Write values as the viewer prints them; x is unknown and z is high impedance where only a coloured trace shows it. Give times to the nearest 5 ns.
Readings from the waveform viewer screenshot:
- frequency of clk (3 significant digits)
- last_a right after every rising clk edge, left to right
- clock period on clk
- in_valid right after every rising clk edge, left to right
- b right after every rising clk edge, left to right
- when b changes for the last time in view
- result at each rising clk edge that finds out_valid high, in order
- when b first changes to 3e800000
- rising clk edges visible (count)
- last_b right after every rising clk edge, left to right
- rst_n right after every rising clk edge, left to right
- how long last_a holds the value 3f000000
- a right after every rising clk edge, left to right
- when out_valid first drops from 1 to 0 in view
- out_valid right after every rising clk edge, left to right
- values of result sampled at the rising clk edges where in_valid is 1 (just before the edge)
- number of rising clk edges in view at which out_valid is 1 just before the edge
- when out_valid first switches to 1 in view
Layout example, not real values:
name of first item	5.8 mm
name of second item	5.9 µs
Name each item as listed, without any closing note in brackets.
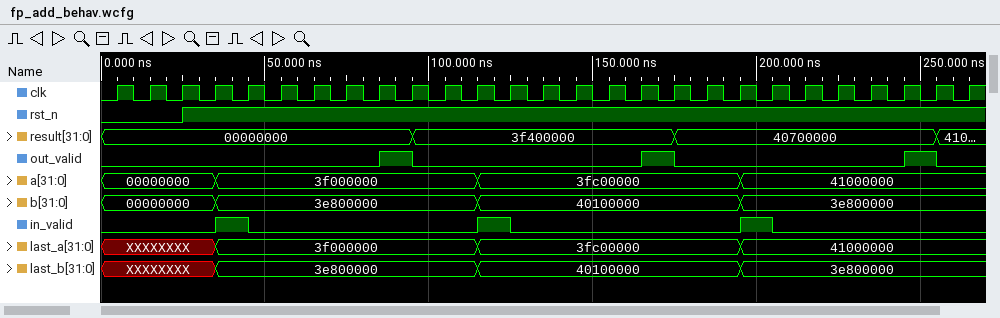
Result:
frequency of clk	100 MHz
last_a right after every rising clk edge, left to right	XXXXXXXX, XXXXXXXX, XXXXXXXX, 3f000000, 3f000000, 3f000000, 3f000000, 3f000000, 3f000000, 3f000000, 3f000000, 3fc00000, 3fc00000, 3fc00000, 3fc00000, 3fc00000, 3fc00000, 3fc00000, 3fc00000, 41000000, 41000000, 41000000, 41000000, 41000000, 41000000, 41000000, 41000000
clock period on clk	10 ns
in_valid right after every rising clk edge, left to right	0 0 0 1 0 0 0 0 0 0 0 1 0 0 0 0 0 0 0 1 0 0 0 0 0 0 0
b right after every rising clk edge, left to right	00000000, 00000000, 00000000, 3e800000, 3e800000, 3e800000, 3e800000, 3e800000, 3e800000, 3e800000, 3e800000, 40100000, 40100000, 40100000, 40100000, 40100000, 40100000, 40100000, 40100000, 3e800000, 3e800000, 3e800000, 3e800000, 3e800000, 3e800000, 3e800000, 3e800000
when b changes for the last time in view	195 ns
result at each rising clk edge that finds out_valid high, in order	00000000, 3f400000, 40700000
when b first changes to 3e800000	35 ns
rising clk edges visible	27
last_b right after every rising clk edge, left to right	XXXXXXXX, XXXXXXXX, XXXXXXXX, 3e800000, 3e800000, 3e800000, 3e800000, 3e800000, 3e800000, 3e800000, 3e800000, 40100000, 40100000, 40100000, 40100000, 40100000, 40100000, 40100000, 40100000, 3e800000, 3e800000, 3e800000, 3e800000, 3e800000, 3e800000, 3e800000, 3e800000
rst_n right after every rising clk edge, left to right	0 0 1 1 1 1 1 1 1 1 1 1 1 1 1 1 1 1 1 1 1 1 1 1 1 1 1
how long last_a holds the value 3f000000	80 ns
a right after every rising clk edge, left to right	00000000, 00000000, 00000000, 3f000000, 3f000000, 3f000000, 3f000000, 3f000000, 3f000000, 3f000000, 3f000000, 3fc00000, 3fc00000, 3fc00000, 3fc00000, 3fc00000, 3fc00000, 3fc00000, 3fc00000, 41000000, 41000000, 41000000, 41000000, 41000000, 41000000, 41000000, 41000000
when out_valid first drops from 1 to 0 in view	95 ns
out_valid right after every rising clk edge, left to right	0 0 0 0 0 0 0 0 1 0 0 0 0 0 0 0 1 0 0 0 0 0 0 0 1 0 0
values of result sampled at the rising clk edges where in_valid is 1	00000000, 3f400000, 40700000
number of rising clk edges in view at which out_valid is 1 just before the edge	3
when out_valid first switches to 1 in view	85 ns
